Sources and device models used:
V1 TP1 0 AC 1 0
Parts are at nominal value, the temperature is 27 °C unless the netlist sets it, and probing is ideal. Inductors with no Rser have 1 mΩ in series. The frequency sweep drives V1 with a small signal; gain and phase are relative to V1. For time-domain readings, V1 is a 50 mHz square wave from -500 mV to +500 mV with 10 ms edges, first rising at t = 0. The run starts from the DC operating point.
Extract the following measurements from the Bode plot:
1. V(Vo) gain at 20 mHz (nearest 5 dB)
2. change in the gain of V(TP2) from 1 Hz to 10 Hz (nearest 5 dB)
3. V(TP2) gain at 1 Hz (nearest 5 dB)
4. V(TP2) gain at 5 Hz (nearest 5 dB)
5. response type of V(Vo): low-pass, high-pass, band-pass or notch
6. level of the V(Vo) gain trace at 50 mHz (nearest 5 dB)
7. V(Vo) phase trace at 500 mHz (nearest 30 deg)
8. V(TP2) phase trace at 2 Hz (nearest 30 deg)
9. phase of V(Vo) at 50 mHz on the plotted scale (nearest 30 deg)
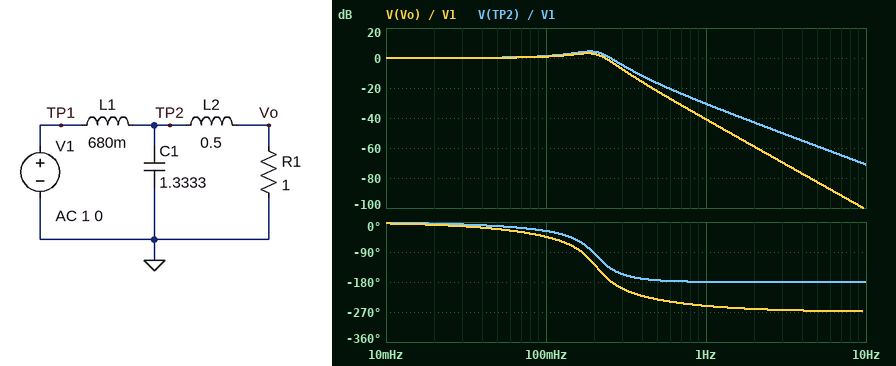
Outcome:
0 dB
-40 dB
-30 dB
-60 dB
low-pass
0 dB
-240 deg
-180 deg
-30 deg
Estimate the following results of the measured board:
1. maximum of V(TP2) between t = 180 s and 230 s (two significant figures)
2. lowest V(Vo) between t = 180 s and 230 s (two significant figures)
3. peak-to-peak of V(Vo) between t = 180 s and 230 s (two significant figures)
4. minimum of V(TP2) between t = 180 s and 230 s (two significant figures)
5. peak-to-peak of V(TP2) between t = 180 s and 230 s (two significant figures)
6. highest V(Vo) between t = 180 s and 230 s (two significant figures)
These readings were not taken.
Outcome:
810 mV
-750 mV
1.5 V
-810 mV
1.6 V
750 mV
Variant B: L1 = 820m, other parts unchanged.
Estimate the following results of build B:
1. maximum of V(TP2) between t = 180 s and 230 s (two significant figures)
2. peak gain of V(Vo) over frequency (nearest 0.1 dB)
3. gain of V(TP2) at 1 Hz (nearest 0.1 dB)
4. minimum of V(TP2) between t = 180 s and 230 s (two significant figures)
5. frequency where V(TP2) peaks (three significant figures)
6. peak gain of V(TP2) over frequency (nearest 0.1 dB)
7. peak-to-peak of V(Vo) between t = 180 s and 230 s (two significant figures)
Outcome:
770 mV
2.2 dB
-32.2 dB
-770 mV
168 mHz
3.2 dB
1.4 V
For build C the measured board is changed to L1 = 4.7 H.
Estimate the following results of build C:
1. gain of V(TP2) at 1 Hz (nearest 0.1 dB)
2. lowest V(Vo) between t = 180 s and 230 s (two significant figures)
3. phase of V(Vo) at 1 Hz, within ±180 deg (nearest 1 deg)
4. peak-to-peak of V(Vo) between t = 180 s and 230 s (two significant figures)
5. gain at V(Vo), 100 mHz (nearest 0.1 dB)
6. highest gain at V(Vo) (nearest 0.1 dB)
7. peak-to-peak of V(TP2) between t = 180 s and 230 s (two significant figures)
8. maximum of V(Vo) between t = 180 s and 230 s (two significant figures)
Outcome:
-47.5 dB
-410 mV
108 deg
820 mV
-9.2 dB
0 dB
840 mV
410 mV
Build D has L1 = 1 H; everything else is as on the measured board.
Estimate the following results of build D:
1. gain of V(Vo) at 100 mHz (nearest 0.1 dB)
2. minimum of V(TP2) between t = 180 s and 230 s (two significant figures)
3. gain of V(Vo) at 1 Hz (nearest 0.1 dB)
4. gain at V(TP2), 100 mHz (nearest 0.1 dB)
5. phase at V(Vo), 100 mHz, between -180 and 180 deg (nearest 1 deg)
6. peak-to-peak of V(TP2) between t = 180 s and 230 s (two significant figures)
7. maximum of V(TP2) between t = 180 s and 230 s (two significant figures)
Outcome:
0.8 dB
-710 mV
-44.3 dB
1.2 dB
-59 deg
1.4 V
710 mV
